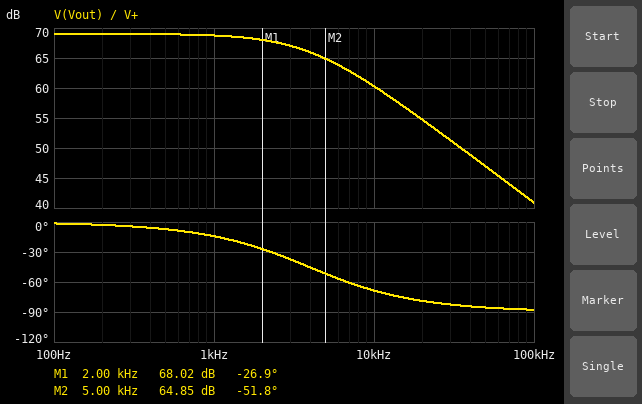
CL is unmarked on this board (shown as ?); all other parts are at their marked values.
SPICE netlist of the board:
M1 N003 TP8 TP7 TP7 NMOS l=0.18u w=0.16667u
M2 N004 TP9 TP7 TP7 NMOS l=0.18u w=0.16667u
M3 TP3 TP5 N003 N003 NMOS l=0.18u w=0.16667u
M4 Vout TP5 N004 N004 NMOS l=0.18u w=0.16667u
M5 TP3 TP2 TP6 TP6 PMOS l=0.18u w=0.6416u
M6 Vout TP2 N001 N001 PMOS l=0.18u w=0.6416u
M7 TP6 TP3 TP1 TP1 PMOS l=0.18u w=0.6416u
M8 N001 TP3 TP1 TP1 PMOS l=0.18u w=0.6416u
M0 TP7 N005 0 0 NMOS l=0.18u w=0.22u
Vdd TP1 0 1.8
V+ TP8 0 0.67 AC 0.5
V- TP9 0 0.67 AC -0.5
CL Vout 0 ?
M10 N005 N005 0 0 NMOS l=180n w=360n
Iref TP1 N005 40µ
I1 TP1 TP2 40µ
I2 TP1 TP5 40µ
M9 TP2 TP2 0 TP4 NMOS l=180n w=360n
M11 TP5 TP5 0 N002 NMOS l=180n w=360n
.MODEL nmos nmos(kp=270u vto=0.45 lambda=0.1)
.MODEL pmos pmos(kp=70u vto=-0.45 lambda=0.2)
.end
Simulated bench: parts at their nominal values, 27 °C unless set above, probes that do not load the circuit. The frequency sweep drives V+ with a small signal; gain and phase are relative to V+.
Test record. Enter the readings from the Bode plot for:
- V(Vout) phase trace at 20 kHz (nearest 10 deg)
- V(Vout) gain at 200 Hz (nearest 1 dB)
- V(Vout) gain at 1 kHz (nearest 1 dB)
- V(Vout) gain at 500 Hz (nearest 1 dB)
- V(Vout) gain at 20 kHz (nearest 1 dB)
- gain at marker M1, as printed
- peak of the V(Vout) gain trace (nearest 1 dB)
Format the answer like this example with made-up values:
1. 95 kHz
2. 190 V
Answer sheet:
1. -80 deg
2. 69 dB
3. 69 dB
4. 69 dB
5. 55 dB
6. 68.02 dB
7. 69 dB
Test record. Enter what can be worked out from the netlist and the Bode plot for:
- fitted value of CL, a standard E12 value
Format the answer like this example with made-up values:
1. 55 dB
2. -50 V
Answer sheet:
1. 820 fF
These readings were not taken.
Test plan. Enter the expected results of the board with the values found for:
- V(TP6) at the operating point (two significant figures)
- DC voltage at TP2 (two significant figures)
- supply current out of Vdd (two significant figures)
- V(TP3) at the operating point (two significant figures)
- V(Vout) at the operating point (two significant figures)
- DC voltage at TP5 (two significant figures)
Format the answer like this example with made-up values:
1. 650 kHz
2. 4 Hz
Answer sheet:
1. 1.4 V
2. 820 mV
3. 130 µA
4. 1.2 V
5. 1.2 V
6. 820 mV
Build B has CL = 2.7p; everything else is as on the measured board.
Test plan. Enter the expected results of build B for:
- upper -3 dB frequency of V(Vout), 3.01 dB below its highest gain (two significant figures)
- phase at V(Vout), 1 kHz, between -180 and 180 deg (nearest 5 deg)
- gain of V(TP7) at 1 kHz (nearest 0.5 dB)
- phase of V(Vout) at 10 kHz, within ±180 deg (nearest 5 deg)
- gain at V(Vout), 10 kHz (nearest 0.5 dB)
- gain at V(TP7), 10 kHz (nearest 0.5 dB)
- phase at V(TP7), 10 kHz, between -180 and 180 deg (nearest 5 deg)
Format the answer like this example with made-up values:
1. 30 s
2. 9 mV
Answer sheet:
1. 1.2 kHz
2. -40 deg
3. -13.0 dB
4. -85 deg
5. 50.5 dB
6. -19.5 dB
7. -10 deg
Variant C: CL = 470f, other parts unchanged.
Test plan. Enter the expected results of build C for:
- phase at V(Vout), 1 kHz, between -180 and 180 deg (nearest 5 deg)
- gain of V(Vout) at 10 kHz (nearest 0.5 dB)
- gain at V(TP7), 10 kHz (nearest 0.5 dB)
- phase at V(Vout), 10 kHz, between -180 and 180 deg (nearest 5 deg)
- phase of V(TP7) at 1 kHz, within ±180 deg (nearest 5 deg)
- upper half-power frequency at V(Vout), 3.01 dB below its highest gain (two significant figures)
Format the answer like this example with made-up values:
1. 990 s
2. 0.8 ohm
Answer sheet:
1. -10 deg
2. 64.0 dB
3. -15.0 dB
4. -55 deg
5. -5 deg
6. 6.9 kHz
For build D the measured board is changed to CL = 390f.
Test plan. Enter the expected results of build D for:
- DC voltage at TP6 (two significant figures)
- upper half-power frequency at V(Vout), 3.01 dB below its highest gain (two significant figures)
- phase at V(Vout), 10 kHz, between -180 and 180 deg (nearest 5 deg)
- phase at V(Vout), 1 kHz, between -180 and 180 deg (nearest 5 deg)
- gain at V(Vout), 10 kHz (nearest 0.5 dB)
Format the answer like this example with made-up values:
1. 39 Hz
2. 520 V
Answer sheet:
1. 1.4 V
2. 8.3 kHz
3. -50 deg
4. -5 deg
5. 65.0 dB
